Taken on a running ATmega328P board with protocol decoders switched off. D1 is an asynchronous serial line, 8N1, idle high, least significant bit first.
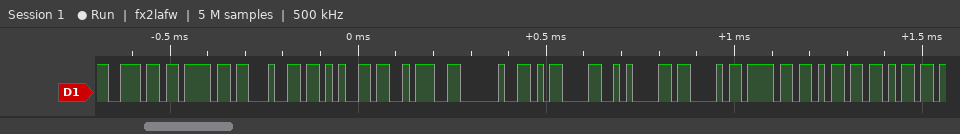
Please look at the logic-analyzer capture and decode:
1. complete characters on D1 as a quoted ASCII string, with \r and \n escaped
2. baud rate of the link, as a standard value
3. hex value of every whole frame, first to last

"node: \r\nComm"
57600 baud
0x6E 0x6F 0x64 0x65 0x3A 0x20 0x0D 0x0A 0x43 0x6F 0x6D 0x6D
